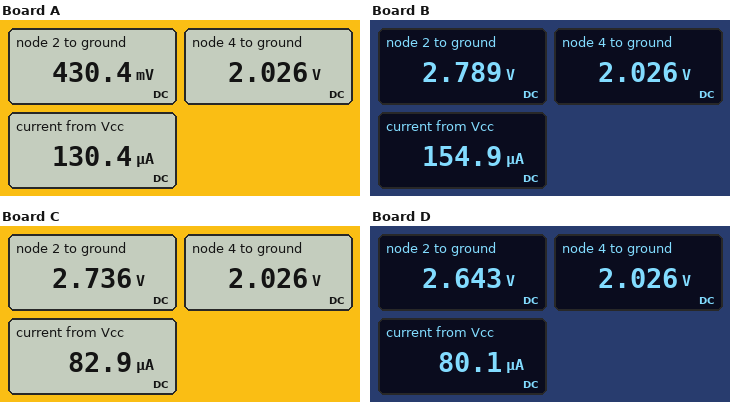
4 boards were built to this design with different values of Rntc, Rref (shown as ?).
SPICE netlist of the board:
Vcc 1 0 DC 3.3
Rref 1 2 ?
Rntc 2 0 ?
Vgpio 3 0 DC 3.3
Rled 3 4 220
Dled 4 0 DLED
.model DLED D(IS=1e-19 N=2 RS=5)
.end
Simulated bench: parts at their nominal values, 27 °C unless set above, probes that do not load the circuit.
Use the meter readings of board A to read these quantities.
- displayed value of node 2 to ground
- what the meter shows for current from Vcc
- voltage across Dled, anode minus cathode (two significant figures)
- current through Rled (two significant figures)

430.4 mV
130.4 µA
2.0 V
5.8 mA
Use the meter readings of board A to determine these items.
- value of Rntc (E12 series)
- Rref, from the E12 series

3.3 kΩ
22 kΩ
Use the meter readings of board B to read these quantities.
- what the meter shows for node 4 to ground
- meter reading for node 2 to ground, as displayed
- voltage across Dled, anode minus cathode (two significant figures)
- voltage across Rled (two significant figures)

2.026 V
2.789 V
2.0 V
1.3 V
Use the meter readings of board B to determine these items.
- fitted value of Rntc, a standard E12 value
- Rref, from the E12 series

18 kΩ
3.3 kΩ
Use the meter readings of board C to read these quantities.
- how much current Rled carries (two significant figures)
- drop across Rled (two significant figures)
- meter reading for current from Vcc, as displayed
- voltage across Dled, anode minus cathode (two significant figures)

5.8 mA
1.3 V
82.9 µA
2.0 V
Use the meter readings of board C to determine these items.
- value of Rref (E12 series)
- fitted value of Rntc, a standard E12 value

6.8 kΩ
33 kΩ
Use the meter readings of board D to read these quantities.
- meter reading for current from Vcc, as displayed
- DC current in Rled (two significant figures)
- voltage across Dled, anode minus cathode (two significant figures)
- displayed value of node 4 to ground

80.1 µA
5.8 mA
2.0 V
2.026 V
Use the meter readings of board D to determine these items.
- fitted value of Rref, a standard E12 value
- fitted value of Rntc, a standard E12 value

8.2 kΩ
33 kΩ
